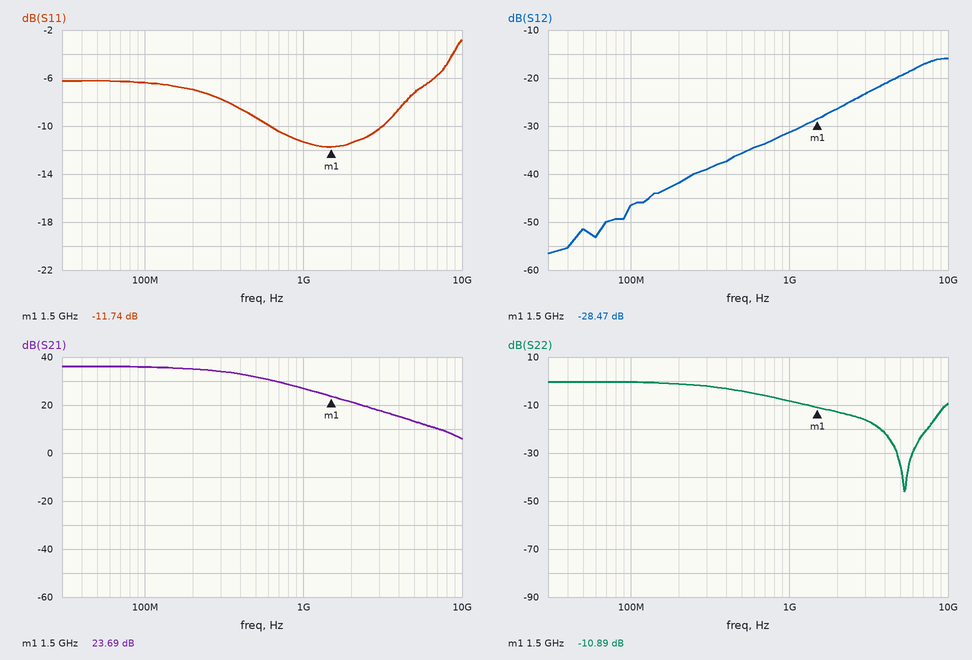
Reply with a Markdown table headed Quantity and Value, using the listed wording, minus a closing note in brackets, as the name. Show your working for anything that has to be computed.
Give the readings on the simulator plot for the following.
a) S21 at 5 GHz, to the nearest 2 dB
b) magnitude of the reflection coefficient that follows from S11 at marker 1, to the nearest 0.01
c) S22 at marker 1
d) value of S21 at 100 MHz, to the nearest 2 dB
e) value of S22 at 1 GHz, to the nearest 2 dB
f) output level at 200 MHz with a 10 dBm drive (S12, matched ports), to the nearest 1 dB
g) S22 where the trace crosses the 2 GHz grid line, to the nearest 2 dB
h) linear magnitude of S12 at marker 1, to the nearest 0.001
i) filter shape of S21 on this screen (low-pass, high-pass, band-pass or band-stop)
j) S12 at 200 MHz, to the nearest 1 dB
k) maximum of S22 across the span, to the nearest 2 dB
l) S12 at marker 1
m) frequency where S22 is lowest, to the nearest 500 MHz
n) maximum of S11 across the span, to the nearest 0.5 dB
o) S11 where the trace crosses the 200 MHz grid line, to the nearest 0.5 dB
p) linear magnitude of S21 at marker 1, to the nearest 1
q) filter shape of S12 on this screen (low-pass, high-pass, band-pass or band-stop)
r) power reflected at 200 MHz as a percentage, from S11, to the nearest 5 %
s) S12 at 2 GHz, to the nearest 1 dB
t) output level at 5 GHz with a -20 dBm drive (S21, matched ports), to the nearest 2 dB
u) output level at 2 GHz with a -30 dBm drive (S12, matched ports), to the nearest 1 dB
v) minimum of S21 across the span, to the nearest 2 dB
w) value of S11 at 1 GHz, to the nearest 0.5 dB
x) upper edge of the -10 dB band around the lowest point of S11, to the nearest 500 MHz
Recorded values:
| Quantity | Value |
|---|---|
| S21 at 5 GHz, to the nearest 2 dB | 14 dB |
| magnitude of the reflection coefficient that follows from S11 at marker 1, to the nearest 0.01 | 10^(-11.74/20) ≈ 0.26 |
| S22 at marker 1 | -10.89 dB |
| value of S21 at 100 MHz, to the nearest 2 dB | 36 dB |
| value of S22 at 1 GHz, to the nearest 2 dB | -8 dB |
| output level at 200 MHz with a 10 dBm drive (S12, matched ports), to the nearest 1 dB | 10 dBm + (-42 dB) = -32 dBm |
| S22 where the trace crosses the 2 GHz grid line, to the nearest 2 dB | -12 dB |
| linear magnitude of S12 at marker 1, to the nearest 0.001 | 10^(-28.47/20) ≈ 0.038 |
| filter shape of S21 on this screen | low-pass |
| S12 at 200 MHz, to the nearest 1 dB | -42 dB |
| maximum of S22 across the span, to the nearest 2 dB | 0 dB |
| S12 at marker 1 | -28.47 dB |
| frequency where S22 is lowest, to the nearest 500 MHz | 5.5 GHz |
| maximum of S11 across the span, to the nearest 0.5 dB | -3.0 dB |
| S11 where the trace crosses the 200 MHz grid line, to the nearest 0.5 dB | -7.0 dB |
| linear magnitude of S21 at marker 1, to the nearest 1 | 10^(23.69/20) ≈ 15 |
| filter shape of S12 on this screen | high-pass |
| power reflected at 200 MHz as a percentage, from S11, to the nearest 5 % | 10^(-7/10) ≈ 20 % |
| S12 at 2 GHz, to the nearest 1 dB | -26 dB |
| output level at 5 GHz with a -20 dBm drive (S21, matched ports), to the nearest 2 dB | -20 dBm + (14 dB) = -6 dBm |
| output level at 2 GHz with a -30 dBm drive (S12, matched ports), to the nearest 1 dB | -30 dBm + (-26 dB) = -56 dBm |
| minimum of S21 across the span, to the nearest 2 dB | 6 dB |
| value of S11 at 1 GHz, to the nearest 0.5 dB | -11.5 dB |
| upper edge of the -10 dB band around the lowest point of S11, to the nearest 500 MHz | 3.0 GHz |
